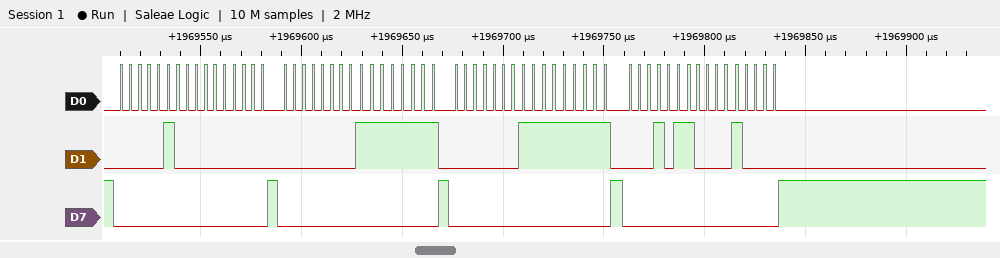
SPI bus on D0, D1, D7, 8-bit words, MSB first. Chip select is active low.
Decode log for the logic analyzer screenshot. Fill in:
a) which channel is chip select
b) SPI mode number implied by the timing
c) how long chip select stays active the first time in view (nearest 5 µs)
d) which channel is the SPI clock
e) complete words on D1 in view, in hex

D7
1
75 µs
D0
04, 00, 00, FF, 01, FF, 16, 10
